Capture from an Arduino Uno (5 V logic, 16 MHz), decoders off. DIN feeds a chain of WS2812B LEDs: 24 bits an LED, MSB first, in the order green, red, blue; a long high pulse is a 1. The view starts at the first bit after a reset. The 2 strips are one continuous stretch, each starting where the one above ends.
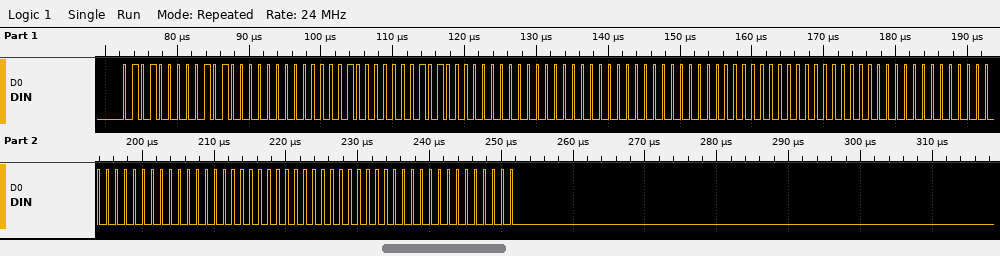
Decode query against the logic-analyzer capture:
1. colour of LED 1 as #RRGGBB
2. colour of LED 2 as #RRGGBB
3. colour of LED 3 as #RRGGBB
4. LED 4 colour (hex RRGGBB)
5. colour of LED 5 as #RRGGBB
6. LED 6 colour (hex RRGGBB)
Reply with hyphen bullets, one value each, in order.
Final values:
- #505000
- #504000
- #000000
- #000000
- #000000
- #000000
